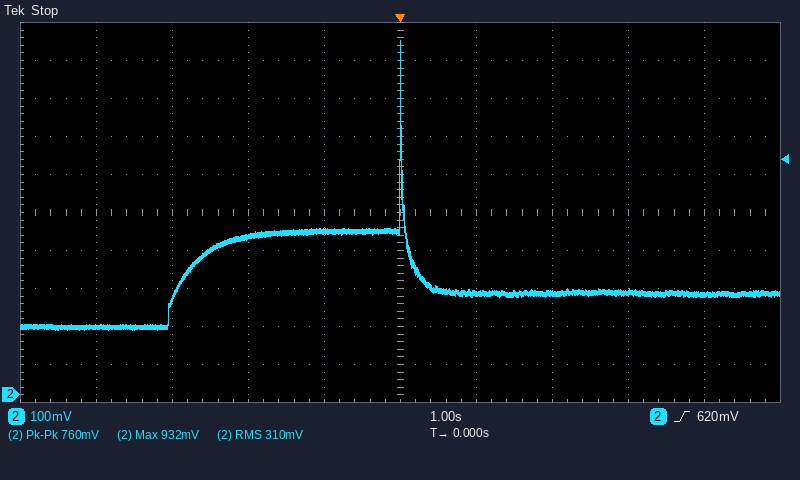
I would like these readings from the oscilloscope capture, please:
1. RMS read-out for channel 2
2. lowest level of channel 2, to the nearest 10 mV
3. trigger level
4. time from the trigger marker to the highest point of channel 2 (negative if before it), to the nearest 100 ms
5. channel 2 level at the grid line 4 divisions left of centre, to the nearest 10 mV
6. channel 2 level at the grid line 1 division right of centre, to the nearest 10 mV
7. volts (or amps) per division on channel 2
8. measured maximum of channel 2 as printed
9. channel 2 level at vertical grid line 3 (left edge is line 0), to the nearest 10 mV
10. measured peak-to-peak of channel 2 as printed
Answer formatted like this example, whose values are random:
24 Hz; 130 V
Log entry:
310 mV; 170 mV; 620 mV; 0.0 s; 180 mV; 270 mV; 100 mV; 932 mV; 420 mV; 760 mV
